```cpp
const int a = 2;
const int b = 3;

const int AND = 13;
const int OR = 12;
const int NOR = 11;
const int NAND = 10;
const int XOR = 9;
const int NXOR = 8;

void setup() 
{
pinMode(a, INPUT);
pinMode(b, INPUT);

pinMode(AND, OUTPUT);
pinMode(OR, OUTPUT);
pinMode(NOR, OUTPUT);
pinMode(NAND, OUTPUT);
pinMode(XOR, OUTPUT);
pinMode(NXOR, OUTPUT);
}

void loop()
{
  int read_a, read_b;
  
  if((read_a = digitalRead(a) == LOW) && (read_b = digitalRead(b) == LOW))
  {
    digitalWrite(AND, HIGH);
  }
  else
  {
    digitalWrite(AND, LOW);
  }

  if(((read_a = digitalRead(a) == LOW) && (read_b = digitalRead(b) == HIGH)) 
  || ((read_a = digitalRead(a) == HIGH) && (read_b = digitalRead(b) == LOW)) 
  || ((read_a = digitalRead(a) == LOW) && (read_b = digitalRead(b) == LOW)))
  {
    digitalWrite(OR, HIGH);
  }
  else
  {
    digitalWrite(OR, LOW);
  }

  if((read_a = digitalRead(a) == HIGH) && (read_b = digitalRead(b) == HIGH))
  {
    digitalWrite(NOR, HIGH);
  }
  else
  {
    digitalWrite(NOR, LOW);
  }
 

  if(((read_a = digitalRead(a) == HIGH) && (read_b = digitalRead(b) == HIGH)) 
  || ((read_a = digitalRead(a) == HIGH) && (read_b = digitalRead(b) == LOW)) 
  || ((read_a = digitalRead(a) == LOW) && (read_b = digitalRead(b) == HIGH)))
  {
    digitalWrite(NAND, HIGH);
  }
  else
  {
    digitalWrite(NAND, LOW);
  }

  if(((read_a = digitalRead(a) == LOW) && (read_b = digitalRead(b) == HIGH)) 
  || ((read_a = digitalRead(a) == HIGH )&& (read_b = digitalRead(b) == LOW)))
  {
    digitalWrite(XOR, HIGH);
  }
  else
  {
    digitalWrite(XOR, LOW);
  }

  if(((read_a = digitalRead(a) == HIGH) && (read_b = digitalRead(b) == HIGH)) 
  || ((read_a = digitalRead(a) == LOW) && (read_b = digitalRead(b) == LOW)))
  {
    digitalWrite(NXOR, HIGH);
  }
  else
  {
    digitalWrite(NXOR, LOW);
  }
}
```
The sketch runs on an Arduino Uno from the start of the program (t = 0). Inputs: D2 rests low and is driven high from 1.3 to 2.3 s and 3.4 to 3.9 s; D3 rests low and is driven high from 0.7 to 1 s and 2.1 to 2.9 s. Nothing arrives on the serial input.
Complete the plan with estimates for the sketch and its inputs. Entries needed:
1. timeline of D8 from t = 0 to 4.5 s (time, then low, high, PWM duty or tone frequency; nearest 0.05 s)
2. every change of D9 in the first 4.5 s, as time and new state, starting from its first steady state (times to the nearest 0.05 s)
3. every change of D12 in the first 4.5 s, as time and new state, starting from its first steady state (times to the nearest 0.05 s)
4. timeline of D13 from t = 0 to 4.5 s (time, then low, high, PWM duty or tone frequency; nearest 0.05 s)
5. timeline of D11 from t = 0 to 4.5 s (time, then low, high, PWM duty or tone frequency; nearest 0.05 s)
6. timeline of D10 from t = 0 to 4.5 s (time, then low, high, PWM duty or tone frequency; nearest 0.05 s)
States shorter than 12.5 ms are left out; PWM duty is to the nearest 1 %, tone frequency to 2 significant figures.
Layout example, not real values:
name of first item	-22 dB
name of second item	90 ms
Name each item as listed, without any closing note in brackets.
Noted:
timeline of D8 from t = 0 to 4.5 s	0 s high; 0.7 s low; 1 s high; 1.3 s low; 2.1 s high; 2.3 s low; 2.9 s high; 3.4 s low; 3.9 s high
every change of D9 in the first 4.5 s, as time and new state, starting from its first steady state	0 s low; 0.7 s high; 1 s low; 1.3 s high; 2.1 s low; 2.3 s high; 2.9 s low; 3.4 s high; 3.9 s low
every change of D12 in the first 4.5 s, as time and new state, starting from its first steady state	0 s high; 2.1 s low; 2.3 s high
timeline of D13 from t = 0 to 4.5 s	0 s high; 0.7 s low; 1 s high; 1.3 s low; 2.9 s high; 3.4 s low; 3.9 s high
timeline of D11 from t = 0 to 4.5 s	0 s low; 2.1 s high; 2.3 s low
timeline of D10 from t = 0 to 4.5 s	0 s low; 0.7 s high; 1 s low; 1.3 s high; 2.9 s low; 3.4 s high; 3.9 s low
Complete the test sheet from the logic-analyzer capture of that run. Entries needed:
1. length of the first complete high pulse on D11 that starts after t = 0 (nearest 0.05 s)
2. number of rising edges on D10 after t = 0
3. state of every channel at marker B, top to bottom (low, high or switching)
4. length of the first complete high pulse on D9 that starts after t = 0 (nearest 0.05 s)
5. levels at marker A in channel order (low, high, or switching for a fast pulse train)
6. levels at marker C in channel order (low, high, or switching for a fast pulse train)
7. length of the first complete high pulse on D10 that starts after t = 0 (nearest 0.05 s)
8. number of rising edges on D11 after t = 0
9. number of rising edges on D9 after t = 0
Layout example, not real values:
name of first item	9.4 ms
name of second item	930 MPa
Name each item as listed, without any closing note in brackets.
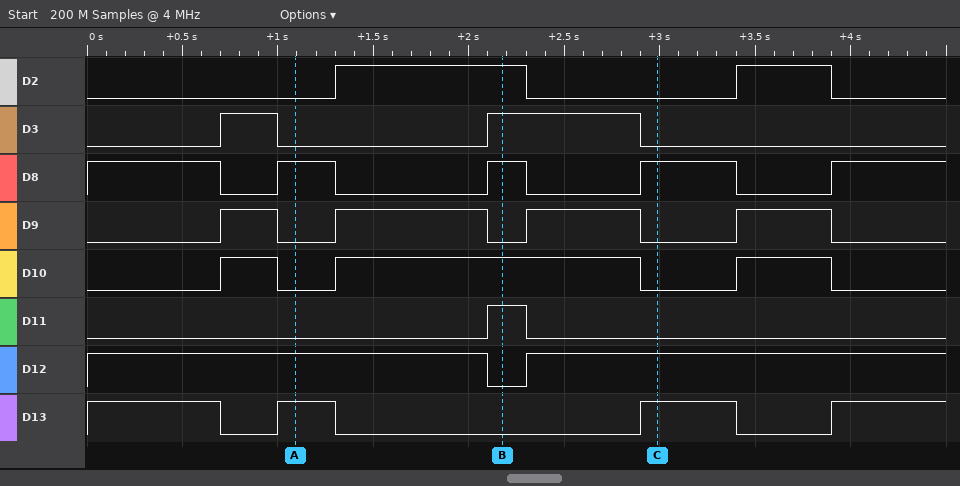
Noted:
length of the first complete high pulse on D11 that starts after t = 0	0.20 s
number of rising edges on D10 after t = 0	3
state of every channel at marker B, top to bottom	D2 high, D3 high, D8 high, D9 low, D10 high, D11 high, D12 low, D13 low
length of the first complete high pulse on D9 that starts after t = 0	0.30 s
levels at marker A in channel order	D2 low, D3 low, D8 high, D9 low, D10 low, D11 low, D12 high, D13 high
levels at marker C in channel order	D2 low, D3 low, D8 high, D9 low, D10 low, D11 low, D12 high, D13 high
length of the first complete high pulse on D10 that starts after t = 0	0.30 s
number of rising edges on D11 after t = 0	1
number of rising edges on D9 after t = 0	4
